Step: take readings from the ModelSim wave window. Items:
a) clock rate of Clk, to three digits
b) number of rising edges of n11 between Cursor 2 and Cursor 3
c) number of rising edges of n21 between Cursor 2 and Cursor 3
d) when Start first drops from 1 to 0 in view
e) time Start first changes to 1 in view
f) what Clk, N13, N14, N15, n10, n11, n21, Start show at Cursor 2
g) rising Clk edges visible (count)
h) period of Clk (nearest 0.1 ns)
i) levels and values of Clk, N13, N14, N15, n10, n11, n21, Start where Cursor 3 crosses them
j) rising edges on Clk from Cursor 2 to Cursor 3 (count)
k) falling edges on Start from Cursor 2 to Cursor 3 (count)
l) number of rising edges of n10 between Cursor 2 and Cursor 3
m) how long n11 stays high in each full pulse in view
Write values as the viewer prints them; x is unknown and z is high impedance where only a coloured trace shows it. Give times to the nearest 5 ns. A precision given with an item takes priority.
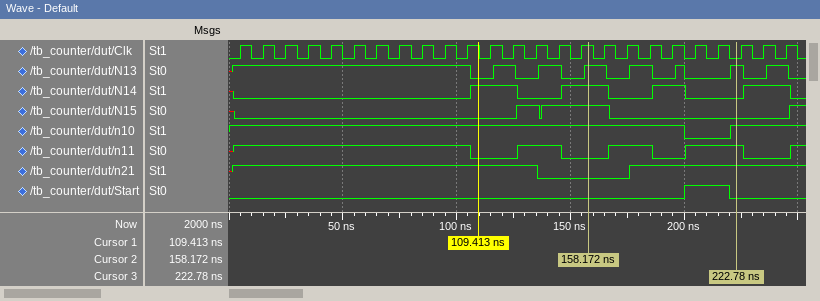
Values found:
100 MHz
2
1
220 ns
200 ns
Clk=1, N13=1, N14=1, N15=1, n10=1, n11=0, n21=0, Start=0
25
10 ns
Clk=0, N13=1, N14=0, N15=0, n10=1, n11=1, n21=1, Start=0
6
1
1
20 ns, 20 ns, 25 ns
